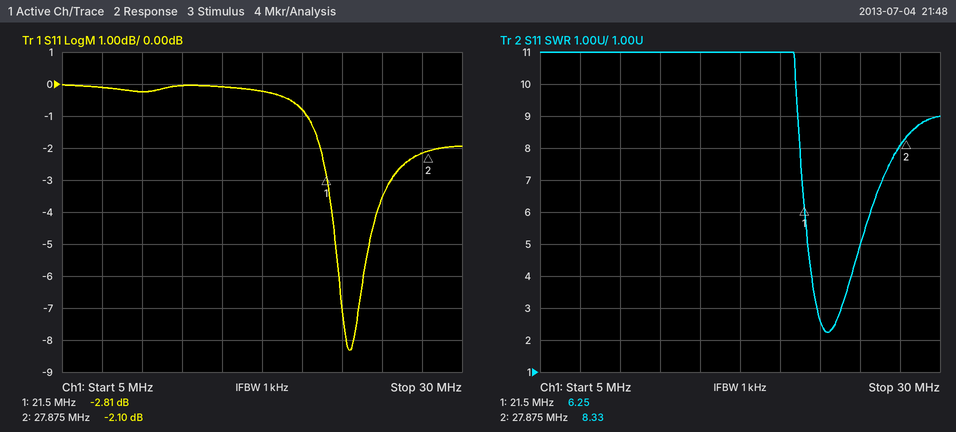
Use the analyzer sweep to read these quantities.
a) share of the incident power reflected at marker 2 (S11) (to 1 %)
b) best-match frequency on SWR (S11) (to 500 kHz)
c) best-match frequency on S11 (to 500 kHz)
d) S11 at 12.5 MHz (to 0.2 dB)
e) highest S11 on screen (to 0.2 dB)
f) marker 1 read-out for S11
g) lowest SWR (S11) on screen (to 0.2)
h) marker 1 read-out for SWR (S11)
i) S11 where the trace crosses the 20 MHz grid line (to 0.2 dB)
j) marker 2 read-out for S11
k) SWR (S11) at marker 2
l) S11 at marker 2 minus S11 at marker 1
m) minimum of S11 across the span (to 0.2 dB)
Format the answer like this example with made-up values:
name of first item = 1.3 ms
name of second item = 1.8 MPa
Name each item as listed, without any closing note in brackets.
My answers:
share of the incident power reflected at marker 2 (S11) = 62 %
best-match frequency on SWR (S11) = 23.0 MHz
best-match frequency on S11 = 23.0 MHz
S11 at 12.5 MHz = 0.0 dB
highest S11 on screen = 0.0 dB
marker 1 read-out for S11 = -2.81 dB
lowest SWR (S11) on screen = 2.2
marker 1 read-out for SWR = 6.25
S11 where the trace crosses the 20 MHz grid line = -0.8 dB
marker 2 read-out for S11 = -2.10 dB
SWR (S11) at marker 2 = 8.33
S11 at marker 2 minus S11 at marker 1 = 0.71 dB
minimum of S11 across the span = -8.4 dB
